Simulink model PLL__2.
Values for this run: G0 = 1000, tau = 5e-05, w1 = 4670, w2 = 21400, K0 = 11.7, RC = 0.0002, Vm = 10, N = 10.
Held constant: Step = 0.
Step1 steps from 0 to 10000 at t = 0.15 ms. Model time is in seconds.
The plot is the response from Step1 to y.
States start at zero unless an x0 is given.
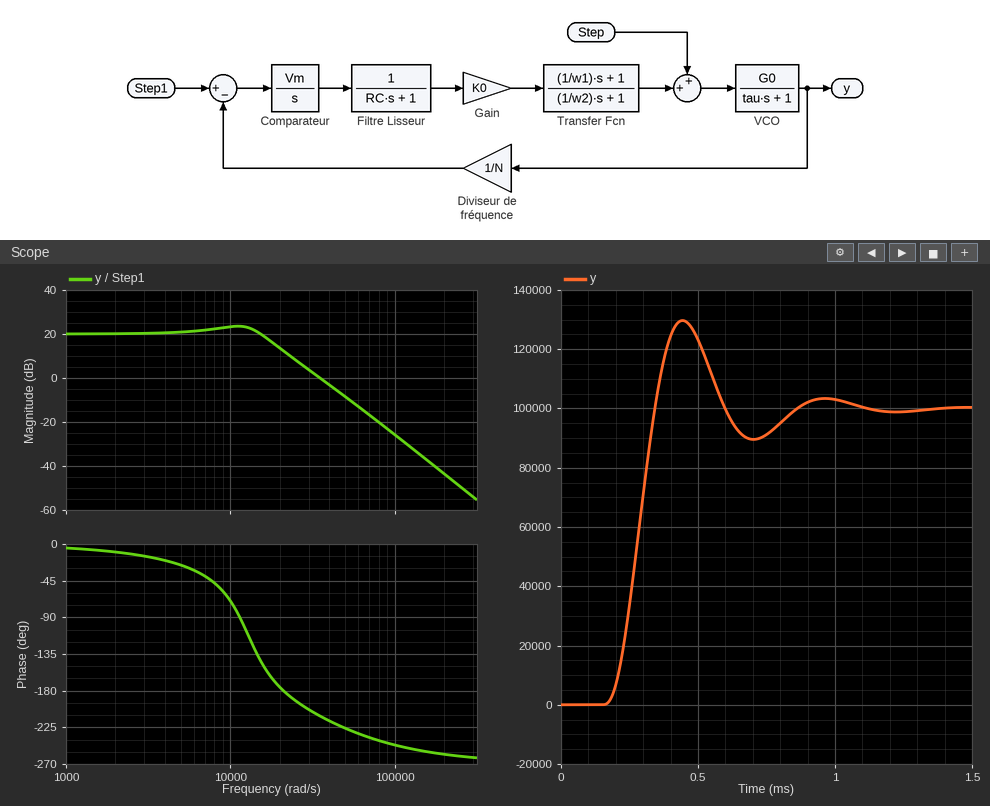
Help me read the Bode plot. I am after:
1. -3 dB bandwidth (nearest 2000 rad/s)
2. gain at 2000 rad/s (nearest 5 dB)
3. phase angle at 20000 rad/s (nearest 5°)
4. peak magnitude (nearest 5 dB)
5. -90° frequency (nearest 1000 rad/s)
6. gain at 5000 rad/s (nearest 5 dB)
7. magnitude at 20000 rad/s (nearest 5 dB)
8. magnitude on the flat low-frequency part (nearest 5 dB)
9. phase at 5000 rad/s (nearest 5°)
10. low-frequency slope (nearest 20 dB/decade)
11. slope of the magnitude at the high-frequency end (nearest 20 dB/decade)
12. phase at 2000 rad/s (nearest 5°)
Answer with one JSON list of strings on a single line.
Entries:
["18000 rad/s", "20 dB", "-175°", "25 dB", "11000 rad/s", "20 dB", "15 dB", "20 dB", "-25°", "0 dB/decade", "-60 dB/decade", "-10°"]
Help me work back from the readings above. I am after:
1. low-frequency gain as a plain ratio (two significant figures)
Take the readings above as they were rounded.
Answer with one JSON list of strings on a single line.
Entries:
["10"]
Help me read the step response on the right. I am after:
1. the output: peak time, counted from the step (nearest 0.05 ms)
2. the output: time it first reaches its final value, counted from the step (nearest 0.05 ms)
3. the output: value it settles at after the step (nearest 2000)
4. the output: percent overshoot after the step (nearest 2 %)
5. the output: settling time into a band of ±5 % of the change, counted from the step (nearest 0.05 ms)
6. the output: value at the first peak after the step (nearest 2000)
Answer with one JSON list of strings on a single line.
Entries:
["0.30 ms", "0.20 ms", "100000", "30 %", "0.65 ms", "130000"]
